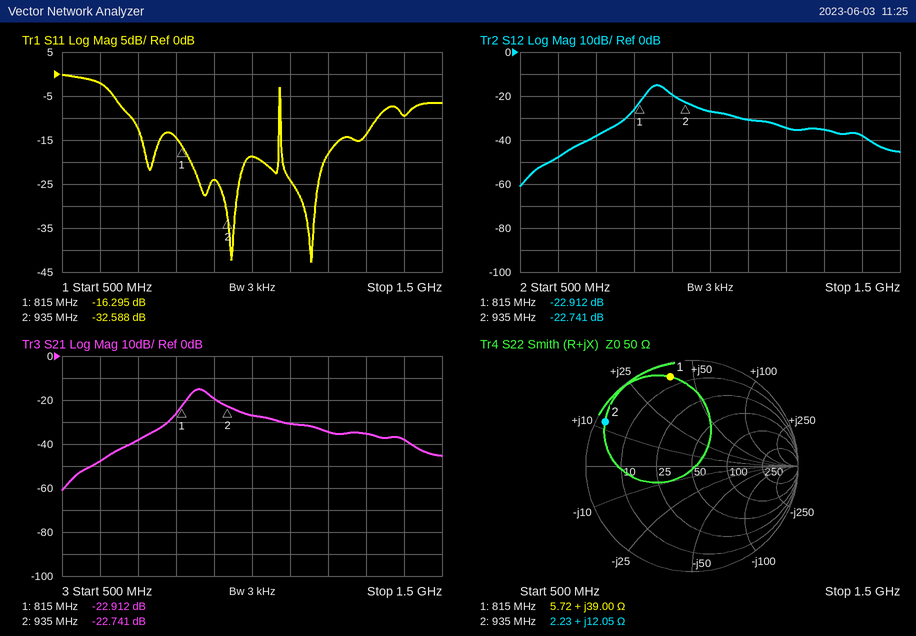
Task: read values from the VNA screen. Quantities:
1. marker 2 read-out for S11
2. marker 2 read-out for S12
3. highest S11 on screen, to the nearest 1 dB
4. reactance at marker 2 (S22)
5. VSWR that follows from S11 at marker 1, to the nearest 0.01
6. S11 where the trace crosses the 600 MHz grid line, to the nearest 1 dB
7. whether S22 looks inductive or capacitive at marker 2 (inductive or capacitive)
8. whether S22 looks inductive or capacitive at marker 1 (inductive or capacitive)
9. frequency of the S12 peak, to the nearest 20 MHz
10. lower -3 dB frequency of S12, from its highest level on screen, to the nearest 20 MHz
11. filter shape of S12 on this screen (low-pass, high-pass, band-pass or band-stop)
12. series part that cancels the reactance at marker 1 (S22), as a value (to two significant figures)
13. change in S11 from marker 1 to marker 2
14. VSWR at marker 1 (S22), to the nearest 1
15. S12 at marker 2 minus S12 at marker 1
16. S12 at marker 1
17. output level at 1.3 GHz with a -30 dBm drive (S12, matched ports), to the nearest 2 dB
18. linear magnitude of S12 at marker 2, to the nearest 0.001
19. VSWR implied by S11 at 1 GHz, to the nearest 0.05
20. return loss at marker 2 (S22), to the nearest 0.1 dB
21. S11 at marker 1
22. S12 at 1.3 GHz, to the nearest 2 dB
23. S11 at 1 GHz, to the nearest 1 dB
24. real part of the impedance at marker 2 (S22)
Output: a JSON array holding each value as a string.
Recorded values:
["-32.588 dB", "-22.741 dB", "0 dB", "+12.05 Ω", "1.36", "-2 dB", "inductive", "inductive", "860 MHz", "840 MHz", "band-pass", "5.0 pF", "-16.293 dB", "14", "0.171 dB", "-22.912 dB", "-66 dBm", "0.073", "1.25", "0.7 dB", "-16.295 dB", "-36 dB", "-19 dB", "2.23 Ω"]
